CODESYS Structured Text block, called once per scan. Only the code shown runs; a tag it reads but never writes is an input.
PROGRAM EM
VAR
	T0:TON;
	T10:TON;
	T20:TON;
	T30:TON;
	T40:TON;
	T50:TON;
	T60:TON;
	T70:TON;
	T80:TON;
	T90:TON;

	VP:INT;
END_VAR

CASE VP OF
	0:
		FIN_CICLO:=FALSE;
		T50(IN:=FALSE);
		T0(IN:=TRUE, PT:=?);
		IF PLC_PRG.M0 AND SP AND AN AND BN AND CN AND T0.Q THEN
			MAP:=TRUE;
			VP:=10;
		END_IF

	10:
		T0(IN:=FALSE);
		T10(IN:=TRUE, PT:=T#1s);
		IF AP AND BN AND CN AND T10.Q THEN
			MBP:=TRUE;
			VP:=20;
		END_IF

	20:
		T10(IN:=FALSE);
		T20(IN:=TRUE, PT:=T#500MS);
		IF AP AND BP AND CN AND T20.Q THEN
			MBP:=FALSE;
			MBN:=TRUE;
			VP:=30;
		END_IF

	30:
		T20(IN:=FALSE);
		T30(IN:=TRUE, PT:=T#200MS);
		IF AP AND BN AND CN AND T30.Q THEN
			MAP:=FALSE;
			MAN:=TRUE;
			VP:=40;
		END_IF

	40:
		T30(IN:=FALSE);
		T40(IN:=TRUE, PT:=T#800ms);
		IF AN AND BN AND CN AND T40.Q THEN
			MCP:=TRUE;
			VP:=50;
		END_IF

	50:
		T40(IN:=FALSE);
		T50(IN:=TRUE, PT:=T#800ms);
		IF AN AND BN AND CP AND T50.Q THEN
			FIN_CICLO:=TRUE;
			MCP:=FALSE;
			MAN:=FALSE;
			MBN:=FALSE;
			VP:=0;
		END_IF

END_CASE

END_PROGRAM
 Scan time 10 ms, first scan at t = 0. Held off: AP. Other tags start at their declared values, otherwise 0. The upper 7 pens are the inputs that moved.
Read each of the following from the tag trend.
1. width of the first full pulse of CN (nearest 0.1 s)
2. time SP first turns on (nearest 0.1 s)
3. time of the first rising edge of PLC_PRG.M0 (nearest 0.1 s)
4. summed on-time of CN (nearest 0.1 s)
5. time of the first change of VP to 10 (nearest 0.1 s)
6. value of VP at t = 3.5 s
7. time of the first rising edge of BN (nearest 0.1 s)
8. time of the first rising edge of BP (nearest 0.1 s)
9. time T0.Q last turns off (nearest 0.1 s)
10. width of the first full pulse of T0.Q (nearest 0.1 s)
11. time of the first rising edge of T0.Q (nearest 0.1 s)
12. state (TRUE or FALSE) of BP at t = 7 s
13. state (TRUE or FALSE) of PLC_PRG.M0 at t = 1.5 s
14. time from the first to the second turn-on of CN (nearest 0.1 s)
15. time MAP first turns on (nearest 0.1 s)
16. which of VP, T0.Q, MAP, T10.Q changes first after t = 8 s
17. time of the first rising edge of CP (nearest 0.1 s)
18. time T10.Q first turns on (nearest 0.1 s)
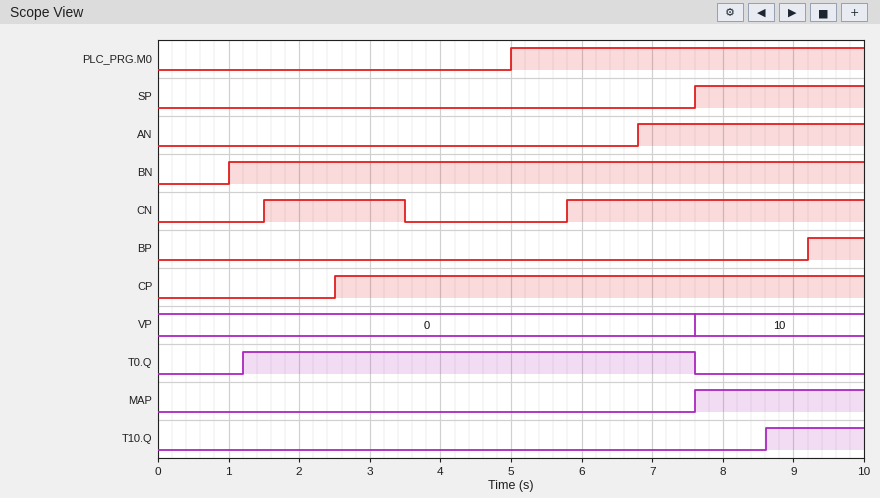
2.0 s
7.6 s
5.0 s
6.2 s
7.6 s
0
1.0 s
9.2 s
7.6 s
6.4 s
1.2 s
FALSE
FALSE
4.3 s
7.6 s
T10.Q
2.5 s
8.6 s
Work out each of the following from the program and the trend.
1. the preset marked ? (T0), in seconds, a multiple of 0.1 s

1.2 s
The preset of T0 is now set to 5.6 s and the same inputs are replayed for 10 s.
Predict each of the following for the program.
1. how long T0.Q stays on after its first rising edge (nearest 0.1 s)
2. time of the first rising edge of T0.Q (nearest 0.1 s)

2.0 s
5.6 s
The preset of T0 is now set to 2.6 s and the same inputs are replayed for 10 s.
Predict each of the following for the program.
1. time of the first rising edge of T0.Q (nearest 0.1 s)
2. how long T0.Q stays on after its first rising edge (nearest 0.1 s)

2.6 s
5.0 s
